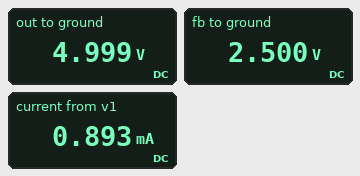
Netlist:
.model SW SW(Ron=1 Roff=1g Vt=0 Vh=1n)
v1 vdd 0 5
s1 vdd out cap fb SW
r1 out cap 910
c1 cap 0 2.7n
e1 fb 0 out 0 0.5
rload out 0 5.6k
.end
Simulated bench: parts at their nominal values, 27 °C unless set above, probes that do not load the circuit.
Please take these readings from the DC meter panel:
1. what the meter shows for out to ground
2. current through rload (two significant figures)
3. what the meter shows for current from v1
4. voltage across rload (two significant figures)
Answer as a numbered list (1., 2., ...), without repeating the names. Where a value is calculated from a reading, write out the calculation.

1. 4.999 V
2. (4.999 V) / 5.6 kΩ = 890 µA
3. 0.893 mA
4. 4.999 V = 5.0 V
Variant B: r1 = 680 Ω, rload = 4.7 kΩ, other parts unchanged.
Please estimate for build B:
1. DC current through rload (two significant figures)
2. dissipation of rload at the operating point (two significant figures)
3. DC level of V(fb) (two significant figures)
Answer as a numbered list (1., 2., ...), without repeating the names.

1. 1.1 mA
2. 5.3 mW
3. 2.5 V
